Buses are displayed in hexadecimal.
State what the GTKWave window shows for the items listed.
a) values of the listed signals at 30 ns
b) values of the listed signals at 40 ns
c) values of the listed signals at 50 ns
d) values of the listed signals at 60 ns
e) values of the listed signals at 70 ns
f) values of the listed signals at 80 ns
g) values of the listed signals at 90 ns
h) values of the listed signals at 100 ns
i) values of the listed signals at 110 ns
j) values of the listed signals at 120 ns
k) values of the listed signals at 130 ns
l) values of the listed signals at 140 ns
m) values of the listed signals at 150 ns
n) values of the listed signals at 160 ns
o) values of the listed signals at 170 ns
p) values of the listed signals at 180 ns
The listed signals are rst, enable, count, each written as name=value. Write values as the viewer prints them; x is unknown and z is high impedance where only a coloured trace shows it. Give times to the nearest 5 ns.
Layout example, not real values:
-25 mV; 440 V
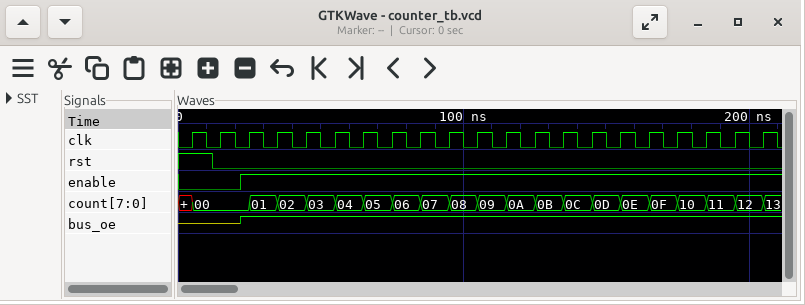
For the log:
rst=0, enable=1, count=01; rst=0, enable=1, count=02; rst=0, enable=1, count=03; rst=0, enable=1, count=04; rst=0, enable=1, count=05; rst=0, enable=1, count=06; rst=0, enable=1, count=07; rst=0, enable=1, count=08; rst=0, enable=1, count=09; rst=0, enable=1, count=0A; rst=0, enable=1, count=0B; rst=0, enable=1, count=0C; rst=0, enable=1, count=0D; rst=0, enable=1, count=0E; rst=0, enable=1, count=0F; rst=0, enable=1, count=10
